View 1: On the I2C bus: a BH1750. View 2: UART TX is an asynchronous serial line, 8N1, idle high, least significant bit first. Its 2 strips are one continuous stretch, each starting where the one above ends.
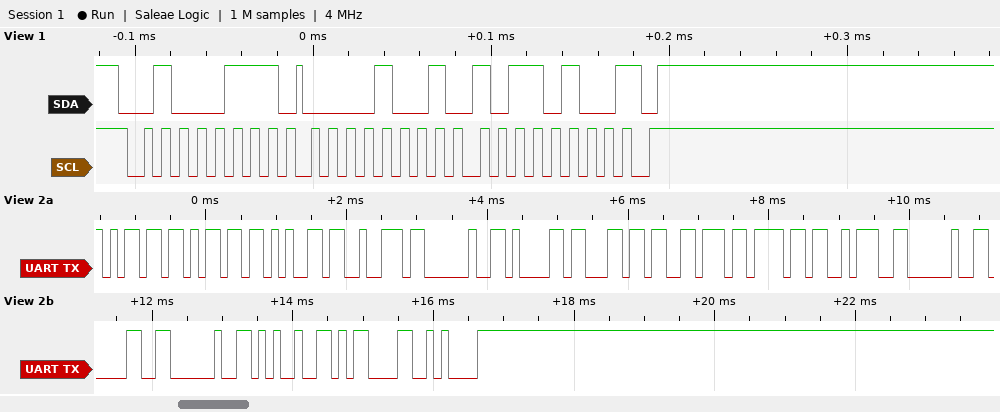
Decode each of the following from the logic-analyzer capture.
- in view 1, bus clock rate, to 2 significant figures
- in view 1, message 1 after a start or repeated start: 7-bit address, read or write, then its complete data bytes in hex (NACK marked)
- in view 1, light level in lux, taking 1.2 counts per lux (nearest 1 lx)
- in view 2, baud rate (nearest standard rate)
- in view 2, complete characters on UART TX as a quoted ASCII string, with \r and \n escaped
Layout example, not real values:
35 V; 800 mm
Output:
100 kHz; 0x23 read: 09 B4 NACK; 2070 lx; 9600 baud; "mmer alvo: 0 %\r\n"
